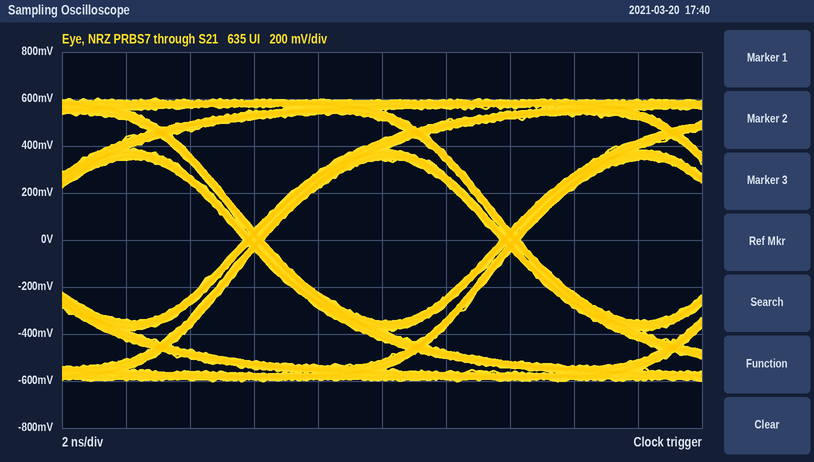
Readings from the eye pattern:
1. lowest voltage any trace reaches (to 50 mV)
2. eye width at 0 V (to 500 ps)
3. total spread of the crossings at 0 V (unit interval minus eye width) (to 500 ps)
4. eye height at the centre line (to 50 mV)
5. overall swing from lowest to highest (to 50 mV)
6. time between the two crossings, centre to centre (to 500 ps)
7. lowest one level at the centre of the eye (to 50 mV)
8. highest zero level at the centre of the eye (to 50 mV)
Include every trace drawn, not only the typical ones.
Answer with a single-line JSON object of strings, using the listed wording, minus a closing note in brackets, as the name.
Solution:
{"lowest voltage any trace reaches": "-600 mV", "eye width at 0 V": "7.5 ns", "total spread of the crossings at 0 V (unit interval minus eye width)": "500 ps", "eye height at the centre line": "700 mV", "overall swing from lowest to highest": "1.20 V", "time between the two crossings, centre to centre": "8.0 ns", "lowest one level at the centre of the eye": "350 mV", "highest zero level at the centre of the eye": "-350 mV"}
